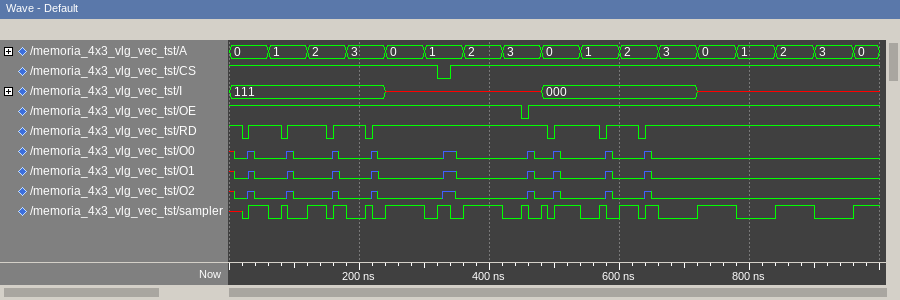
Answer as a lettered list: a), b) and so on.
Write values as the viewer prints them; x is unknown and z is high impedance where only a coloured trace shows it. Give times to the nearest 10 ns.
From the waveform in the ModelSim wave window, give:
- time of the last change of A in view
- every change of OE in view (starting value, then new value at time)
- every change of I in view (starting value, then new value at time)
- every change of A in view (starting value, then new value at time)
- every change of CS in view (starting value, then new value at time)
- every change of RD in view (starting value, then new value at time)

a) 960 ns
b) 1, 0 at 450 ns, 1 at 460 ns
c) 111, x at 240 ns, 000 at 480 ns, x at 720 ns
d) 0, 1 at 60 ns, 2 at 120 ns, 3 at 180 ns, 0 at 240 ns, 1 at 300 ns, 2 at 360 ns, 3 at 420 ns, 0 at 480 ns, 1 at 540 ns, 2 at 600 ns, 3 at 660 ns, 0 at 720 ns, 1 at 780 ns, 2 at 840 ns, 3 at 900 ns, 0 at 960 ns
e) 1, 0 at 320 ns, 1 at 340 ns
f) 1, 0 at 20 ns, 1 at 30 ns, 0 at 80 ns, 1 at 90 ns, 0 at 150 ns, 1 at 160 ns, 0 at 210 ns, 1 at 220 ns, 0 at 490 ns, 1 at 500 ns, 0 at 570 ns, 1 at 580 ns, 0 at 630 ns, 1 at 640 ns
